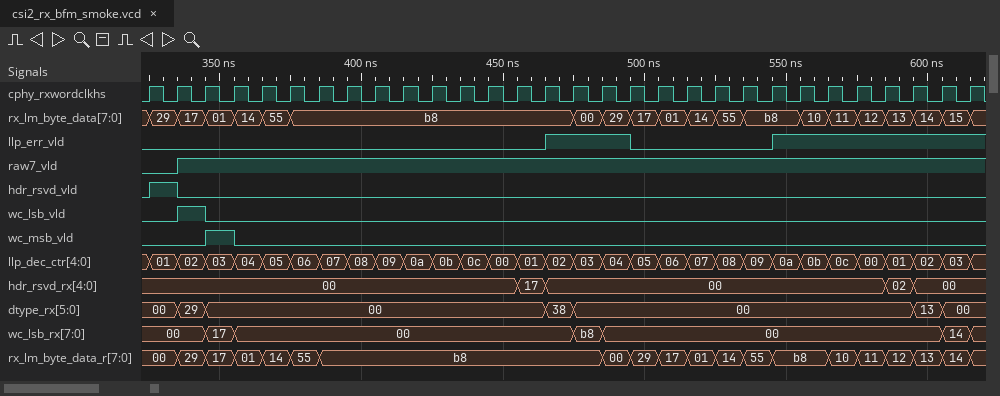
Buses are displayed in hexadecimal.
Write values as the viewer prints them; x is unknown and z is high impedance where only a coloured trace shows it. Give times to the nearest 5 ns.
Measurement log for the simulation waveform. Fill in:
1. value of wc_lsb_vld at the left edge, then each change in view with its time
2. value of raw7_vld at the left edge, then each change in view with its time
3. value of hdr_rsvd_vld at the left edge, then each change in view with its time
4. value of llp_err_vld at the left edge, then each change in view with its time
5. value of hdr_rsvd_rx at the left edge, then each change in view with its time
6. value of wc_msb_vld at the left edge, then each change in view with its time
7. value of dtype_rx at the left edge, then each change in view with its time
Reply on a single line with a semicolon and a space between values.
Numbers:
0, 1 at 335 ns, 0 at 345 ns; 0, 1 at 335 ns; 0, 1 at 325 ns, 0 at 335 ns; 0, 1 at 465 ns, 0 at 495 ns, 1 at 545 ns; 00, 17 at 455 ns, 00 at 465 ns, 02 at 585 ns, 00 at 595 ns; 0, 1 at 345 ns, 0 at 355 ns; 00, 29 at 335 ns, 00 at 345 ns, 38 at 465 ns, 00 at 475 ns, 13 at 595 ns, 00 at 605 ns
